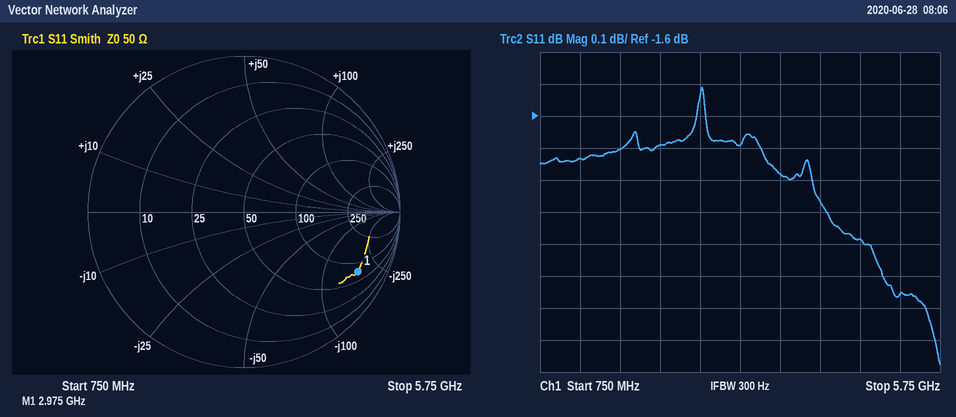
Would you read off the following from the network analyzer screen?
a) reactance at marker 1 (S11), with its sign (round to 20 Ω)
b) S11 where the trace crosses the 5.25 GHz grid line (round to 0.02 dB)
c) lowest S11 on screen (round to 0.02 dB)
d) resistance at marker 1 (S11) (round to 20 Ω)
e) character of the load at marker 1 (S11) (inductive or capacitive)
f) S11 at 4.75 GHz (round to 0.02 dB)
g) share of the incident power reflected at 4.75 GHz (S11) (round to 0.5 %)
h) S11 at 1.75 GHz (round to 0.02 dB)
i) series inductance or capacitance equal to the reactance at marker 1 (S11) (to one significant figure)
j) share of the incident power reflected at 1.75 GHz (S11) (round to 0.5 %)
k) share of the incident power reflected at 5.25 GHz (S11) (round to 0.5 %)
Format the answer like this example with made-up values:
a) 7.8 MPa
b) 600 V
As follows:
a) -180 Ω
b) -2.16 dB
c) -2.38 dB
d) 80 Ω
e) capacitive
f) -1.98 dB
g) 63.5 %
h) -1.70 dB
i) 300 fF
j) 67.5 %
k) 61.0 %
